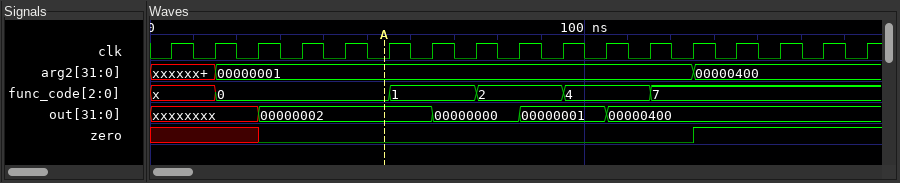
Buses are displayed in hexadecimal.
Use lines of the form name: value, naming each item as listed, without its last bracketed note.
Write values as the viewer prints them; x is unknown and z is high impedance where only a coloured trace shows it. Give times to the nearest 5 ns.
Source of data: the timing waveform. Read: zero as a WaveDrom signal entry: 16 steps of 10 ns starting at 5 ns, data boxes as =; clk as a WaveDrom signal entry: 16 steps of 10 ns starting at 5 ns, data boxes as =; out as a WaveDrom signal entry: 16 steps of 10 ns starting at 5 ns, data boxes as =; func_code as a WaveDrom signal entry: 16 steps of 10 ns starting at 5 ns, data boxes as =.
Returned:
zero as a WaveDrom signal entry: 16 steps of 10 ns starting at 5 ns, data boxes as =: {name: 'zero', wave: 'x.0.........1...'}
clk as a WaveDrom signal entry: 16 steps of 10 ns starting at 5 ns, data boxes as =: {name: 'clk', wave: 'p...............'}
out as a WaveDrom signal entry: 16 steps of 10 ns starting at 5 ns, data boxes as =: {name: 'out', wave: 'x.=...=.=.=.....', data: '00000002 00000000 00000001 00000400'}
func_code as a WaveDrom signal entry: 16 steps of 10 ns starting at 5 ns, data boxes as =: {name: 'func_code', wave: 'x=...=.=.=.=....', data: '0 1 2 4 7'}
